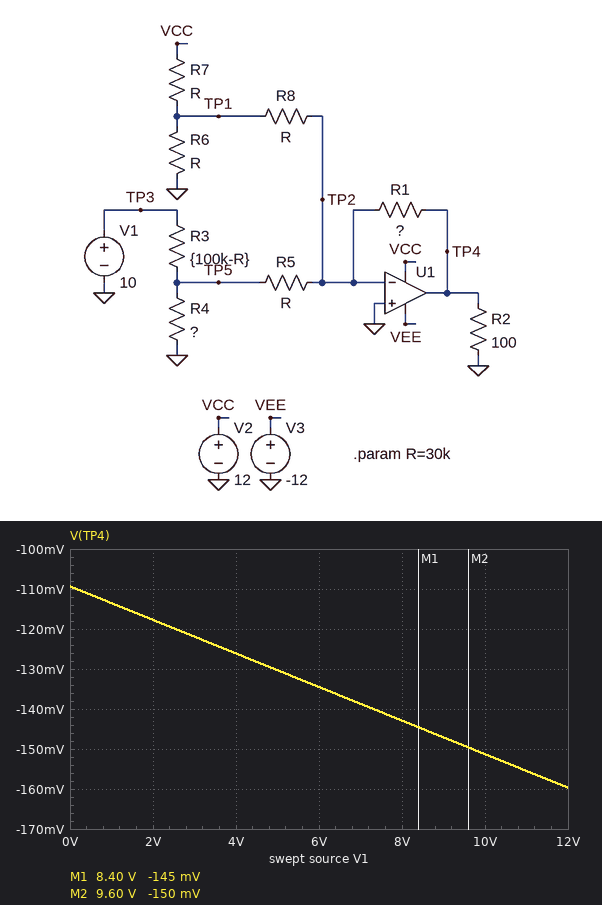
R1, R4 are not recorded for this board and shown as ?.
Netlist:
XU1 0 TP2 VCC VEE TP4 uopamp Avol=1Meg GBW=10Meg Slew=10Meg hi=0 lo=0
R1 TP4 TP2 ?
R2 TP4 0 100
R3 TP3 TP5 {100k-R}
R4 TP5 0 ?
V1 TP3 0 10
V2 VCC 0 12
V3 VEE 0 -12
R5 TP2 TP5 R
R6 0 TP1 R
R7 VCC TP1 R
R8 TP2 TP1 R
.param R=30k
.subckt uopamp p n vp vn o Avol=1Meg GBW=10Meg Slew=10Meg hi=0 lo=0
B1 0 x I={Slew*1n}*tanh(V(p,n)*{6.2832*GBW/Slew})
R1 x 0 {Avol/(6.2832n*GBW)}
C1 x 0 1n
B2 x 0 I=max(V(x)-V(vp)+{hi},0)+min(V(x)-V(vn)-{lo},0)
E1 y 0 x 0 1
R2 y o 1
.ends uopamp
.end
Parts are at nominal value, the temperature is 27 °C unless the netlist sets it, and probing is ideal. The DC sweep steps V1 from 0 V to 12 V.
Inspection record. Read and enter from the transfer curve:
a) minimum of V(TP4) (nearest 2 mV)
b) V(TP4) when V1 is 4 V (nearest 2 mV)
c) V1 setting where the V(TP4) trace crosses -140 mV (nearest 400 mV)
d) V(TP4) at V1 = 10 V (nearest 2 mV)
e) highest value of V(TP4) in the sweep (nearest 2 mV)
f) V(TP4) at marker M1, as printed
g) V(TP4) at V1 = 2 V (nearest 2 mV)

-160 mV
-126 mV
7.2 V
-152 mV
-110 mV
-145 mV
-118 mV
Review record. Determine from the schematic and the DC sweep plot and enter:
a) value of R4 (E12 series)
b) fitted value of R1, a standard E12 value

22 kΩ
820 Ω
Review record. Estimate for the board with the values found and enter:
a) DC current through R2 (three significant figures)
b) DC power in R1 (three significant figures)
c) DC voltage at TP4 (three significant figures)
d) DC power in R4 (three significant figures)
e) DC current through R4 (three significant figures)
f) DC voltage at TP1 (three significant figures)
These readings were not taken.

1.51 mA
27.9 µW
-151 mV
107 µW
69.8 µA
4.00 V
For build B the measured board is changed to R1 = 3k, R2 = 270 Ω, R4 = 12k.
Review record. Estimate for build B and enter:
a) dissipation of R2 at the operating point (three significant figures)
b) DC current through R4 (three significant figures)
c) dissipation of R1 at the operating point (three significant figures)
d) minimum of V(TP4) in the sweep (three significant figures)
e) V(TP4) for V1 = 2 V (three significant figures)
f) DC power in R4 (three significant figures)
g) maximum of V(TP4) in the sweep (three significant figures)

960 µW
90.9 µA
86.4 µW
-531 mV
-422 mV
99.2 µW
-400 mV
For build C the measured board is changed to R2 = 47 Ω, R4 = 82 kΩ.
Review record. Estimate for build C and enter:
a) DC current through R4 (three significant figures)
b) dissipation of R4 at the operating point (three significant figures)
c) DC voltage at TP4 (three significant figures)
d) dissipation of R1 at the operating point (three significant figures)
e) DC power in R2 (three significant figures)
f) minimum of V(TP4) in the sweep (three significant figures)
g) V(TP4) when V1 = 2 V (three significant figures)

29.1 µA
69.6 µW
-175 mV
37.2 µW
649 µW
-188 mV
-122 mV
